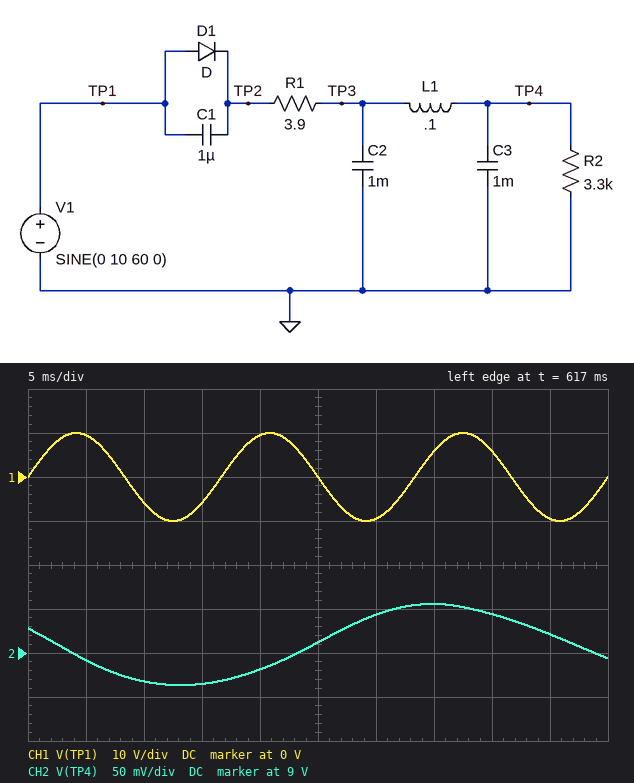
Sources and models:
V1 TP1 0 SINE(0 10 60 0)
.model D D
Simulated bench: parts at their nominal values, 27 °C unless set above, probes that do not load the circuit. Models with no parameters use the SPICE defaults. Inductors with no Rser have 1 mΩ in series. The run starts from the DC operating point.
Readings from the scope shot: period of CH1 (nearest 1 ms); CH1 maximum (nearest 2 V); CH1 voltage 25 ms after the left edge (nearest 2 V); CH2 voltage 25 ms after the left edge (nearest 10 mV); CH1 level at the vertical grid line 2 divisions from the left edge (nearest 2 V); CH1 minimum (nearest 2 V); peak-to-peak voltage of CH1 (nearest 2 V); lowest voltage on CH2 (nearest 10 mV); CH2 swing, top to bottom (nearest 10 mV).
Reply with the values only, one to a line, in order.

17 ms
10 V
0 V
9.01 V
-6 V
-10 V
20 V
8.96 V
90 mV
